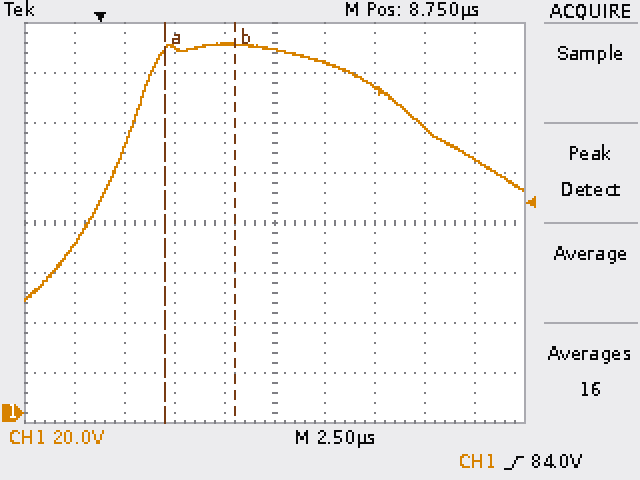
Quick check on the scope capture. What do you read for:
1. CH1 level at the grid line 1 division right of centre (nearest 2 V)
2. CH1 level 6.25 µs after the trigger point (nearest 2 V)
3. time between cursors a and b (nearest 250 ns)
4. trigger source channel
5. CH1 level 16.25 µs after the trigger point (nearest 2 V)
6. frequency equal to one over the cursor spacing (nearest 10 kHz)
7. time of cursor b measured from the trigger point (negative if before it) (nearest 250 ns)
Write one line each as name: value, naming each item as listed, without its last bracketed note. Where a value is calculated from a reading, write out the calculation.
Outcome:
CH1 level at the grid line 1 division right of centre: 140 V
CH1 level 6.25 µs after the trigger point: 148 V
time between cursors a and b: 3.50 µs
trigger source channel: CH1
CH1 level 16.25 µs after the trigger point: 114 V
frequency equal to one over the cursor spacing: 1 / 3.50 µs ≈ 290 kHz
time of cursor b measured from the trigger point (negative if before it): +6.75 µs
